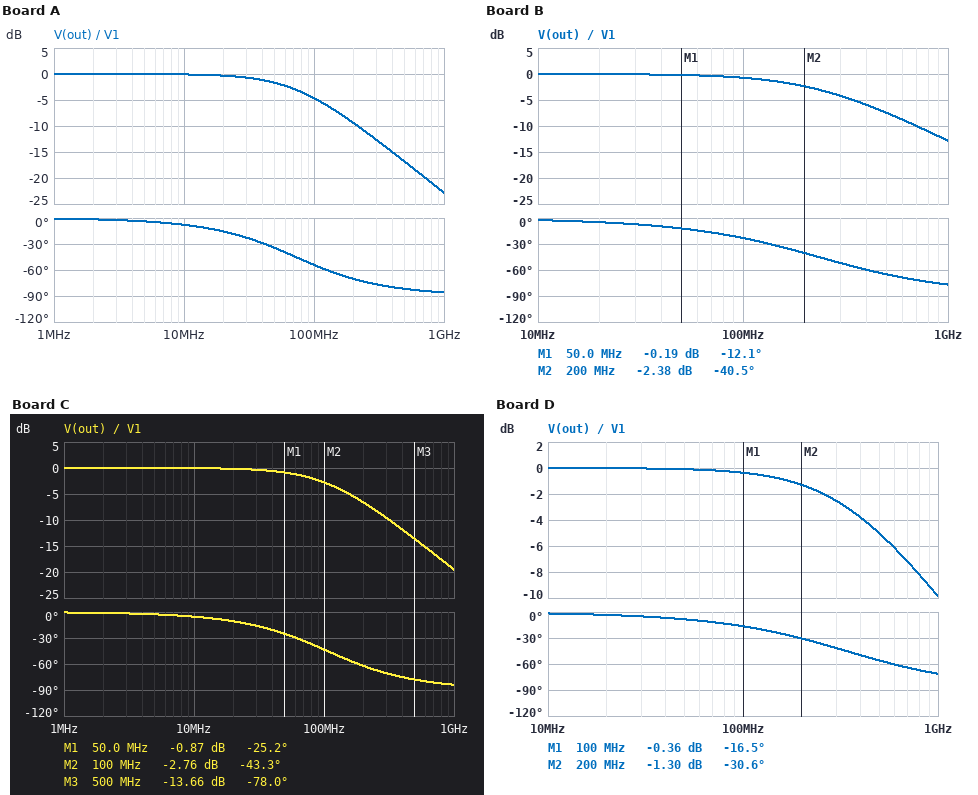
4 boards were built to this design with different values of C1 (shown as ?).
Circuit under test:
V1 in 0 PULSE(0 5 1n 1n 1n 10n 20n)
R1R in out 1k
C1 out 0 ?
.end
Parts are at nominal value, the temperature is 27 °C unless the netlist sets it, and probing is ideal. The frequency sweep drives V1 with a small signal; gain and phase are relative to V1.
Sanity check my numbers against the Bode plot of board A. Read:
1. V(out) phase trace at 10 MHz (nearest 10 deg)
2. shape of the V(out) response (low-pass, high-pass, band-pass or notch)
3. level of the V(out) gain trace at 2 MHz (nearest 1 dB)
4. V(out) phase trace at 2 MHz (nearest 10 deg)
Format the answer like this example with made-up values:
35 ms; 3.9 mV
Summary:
-10 deg; low-pass; 0 dB; 0 deg
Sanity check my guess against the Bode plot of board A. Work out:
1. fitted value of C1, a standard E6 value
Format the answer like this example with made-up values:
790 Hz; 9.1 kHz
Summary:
2.2 pF
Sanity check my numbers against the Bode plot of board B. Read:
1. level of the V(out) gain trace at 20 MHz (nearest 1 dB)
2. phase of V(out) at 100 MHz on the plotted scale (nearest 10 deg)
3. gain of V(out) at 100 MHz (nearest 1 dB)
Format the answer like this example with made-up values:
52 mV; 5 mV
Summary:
0 dB; -20 deg; -1 dB
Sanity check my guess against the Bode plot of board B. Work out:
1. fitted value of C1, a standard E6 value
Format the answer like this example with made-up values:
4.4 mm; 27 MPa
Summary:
680 fF
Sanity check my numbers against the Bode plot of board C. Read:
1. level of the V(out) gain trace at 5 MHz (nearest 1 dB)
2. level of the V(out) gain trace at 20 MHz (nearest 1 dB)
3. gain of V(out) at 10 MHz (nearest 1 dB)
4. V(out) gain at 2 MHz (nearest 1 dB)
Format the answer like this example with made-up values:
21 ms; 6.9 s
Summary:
0 dB; 0 dB; 0 dB; 0 dB
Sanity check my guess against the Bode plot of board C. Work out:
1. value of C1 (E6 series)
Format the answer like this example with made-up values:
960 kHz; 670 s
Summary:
1.5 pF
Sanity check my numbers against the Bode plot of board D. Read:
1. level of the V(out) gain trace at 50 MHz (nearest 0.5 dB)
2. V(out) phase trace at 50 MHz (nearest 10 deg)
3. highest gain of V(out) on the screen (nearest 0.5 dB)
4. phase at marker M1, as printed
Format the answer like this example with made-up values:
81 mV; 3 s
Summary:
0 dB; -10 deg; 0 dB; -16.5 deg
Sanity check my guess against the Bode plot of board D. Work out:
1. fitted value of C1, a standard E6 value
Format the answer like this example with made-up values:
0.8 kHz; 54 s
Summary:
470 fF
